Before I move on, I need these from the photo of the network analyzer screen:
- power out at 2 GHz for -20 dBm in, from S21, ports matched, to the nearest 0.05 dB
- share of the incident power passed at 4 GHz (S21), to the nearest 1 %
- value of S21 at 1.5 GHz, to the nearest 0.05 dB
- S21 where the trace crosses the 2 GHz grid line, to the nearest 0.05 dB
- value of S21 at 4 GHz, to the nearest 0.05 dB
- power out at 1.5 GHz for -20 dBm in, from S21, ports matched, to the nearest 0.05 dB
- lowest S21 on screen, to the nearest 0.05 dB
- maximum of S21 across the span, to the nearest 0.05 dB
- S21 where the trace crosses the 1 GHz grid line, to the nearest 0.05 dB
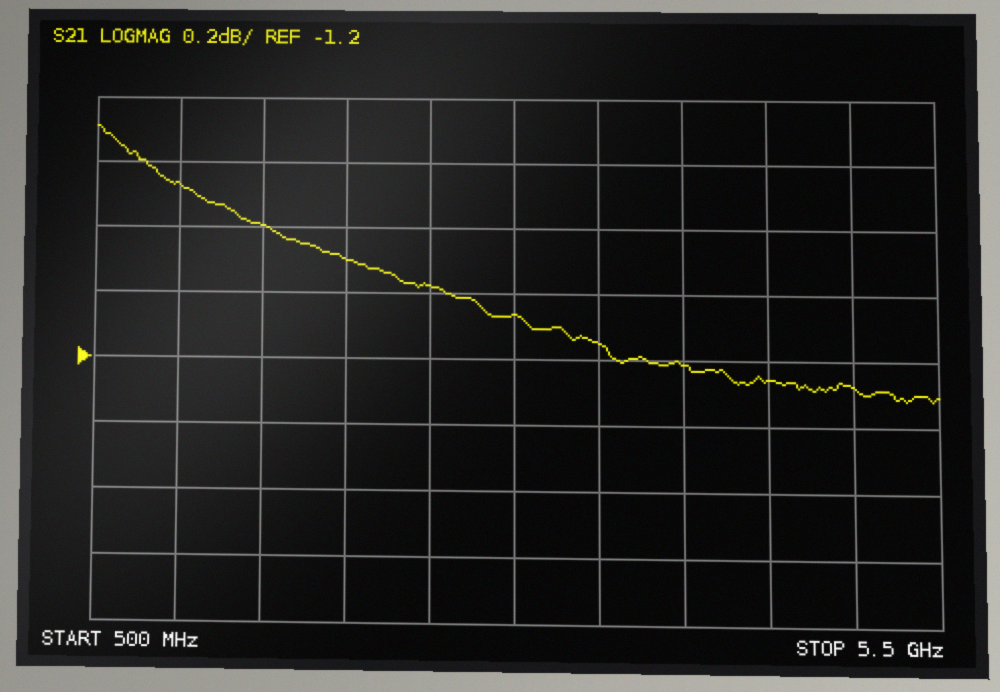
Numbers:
-20.90 dBm
76 %
-0.80 dB
-0.90 dB
-1.20 dB
-20.80 dBm
-1.30 dB
-0.50 dB
-0.65 dB
